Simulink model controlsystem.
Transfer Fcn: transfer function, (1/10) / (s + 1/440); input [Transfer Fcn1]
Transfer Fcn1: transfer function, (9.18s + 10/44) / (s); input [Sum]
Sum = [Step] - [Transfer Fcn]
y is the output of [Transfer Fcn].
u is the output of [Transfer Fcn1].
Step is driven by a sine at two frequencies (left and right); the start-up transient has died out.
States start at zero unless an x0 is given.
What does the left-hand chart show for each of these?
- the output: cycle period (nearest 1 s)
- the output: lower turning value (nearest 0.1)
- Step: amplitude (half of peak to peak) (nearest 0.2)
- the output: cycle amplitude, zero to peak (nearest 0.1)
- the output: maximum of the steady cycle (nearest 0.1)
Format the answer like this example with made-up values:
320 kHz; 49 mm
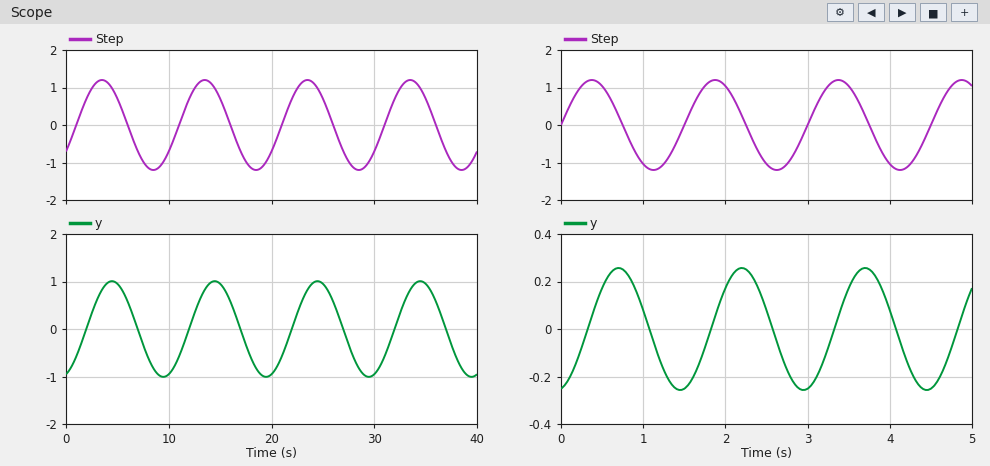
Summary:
10 s; -1.0; 1.2; 1.0; 1.0
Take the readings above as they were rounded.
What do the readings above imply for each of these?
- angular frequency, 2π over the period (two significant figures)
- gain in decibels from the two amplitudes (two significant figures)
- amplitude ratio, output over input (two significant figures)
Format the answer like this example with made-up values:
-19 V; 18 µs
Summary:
0.63 rad/s; -1.6 dB; 0.83
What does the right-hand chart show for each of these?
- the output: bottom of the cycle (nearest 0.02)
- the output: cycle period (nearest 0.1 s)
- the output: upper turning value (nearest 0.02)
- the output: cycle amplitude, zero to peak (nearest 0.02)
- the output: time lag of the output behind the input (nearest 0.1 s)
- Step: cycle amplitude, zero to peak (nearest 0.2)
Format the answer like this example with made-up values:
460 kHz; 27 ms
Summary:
-0.26; 1.5 s; 0.26; 0.26; 0.3 s; 1.2
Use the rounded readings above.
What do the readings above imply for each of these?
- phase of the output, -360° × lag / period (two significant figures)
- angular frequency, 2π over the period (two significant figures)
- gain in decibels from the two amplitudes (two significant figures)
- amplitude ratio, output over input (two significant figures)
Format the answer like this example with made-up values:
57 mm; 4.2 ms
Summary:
-72°; 4.2 rad/s; -13 dB; 0.22
